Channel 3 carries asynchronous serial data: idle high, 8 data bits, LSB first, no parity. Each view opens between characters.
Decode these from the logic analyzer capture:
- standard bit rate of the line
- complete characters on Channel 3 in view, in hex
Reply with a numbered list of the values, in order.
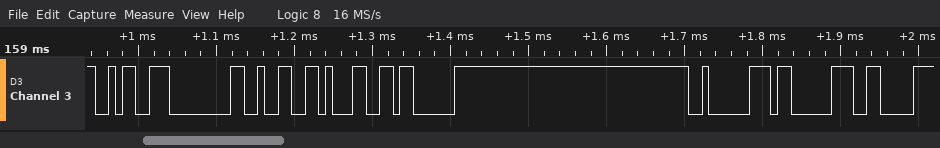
1. 115200 baud
2. 9A, 00, 32, 31, 03, 02, 03, 06
